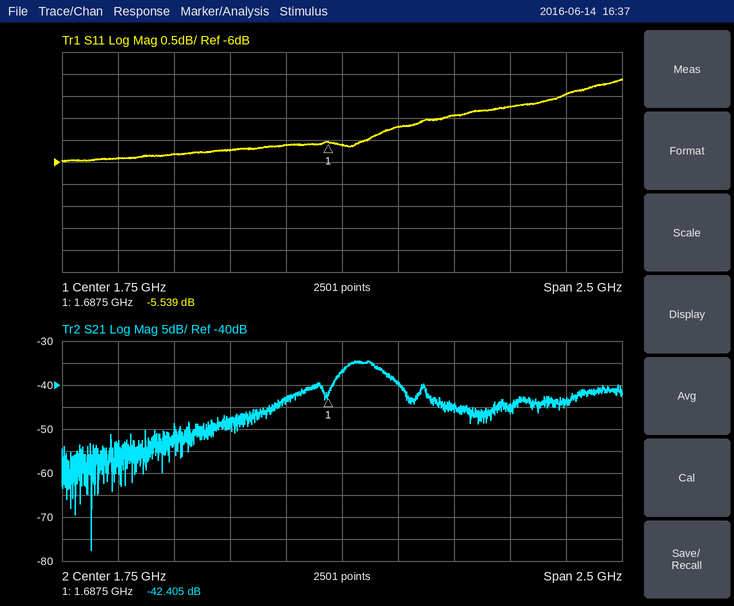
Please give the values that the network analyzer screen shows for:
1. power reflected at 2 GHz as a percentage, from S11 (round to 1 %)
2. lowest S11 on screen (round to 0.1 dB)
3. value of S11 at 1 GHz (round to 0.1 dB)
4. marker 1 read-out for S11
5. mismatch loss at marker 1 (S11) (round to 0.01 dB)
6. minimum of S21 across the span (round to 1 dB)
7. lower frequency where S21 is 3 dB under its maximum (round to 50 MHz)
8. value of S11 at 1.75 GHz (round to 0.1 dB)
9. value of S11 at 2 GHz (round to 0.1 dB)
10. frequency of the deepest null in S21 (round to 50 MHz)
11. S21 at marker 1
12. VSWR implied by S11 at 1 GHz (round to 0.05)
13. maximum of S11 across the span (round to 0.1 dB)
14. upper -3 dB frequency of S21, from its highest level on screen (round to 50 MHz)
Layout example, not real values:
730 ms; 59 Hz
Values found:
30 %; -6.0 dB; -5.8 dB; -5.539 dB; 1.42 dB; -78 dB; 1.75 GHz; -5.6 dB; -5.2 dB; 650 MHz; -42.405 dB; 3.10; -4.1 dB; 1.95 GHz
